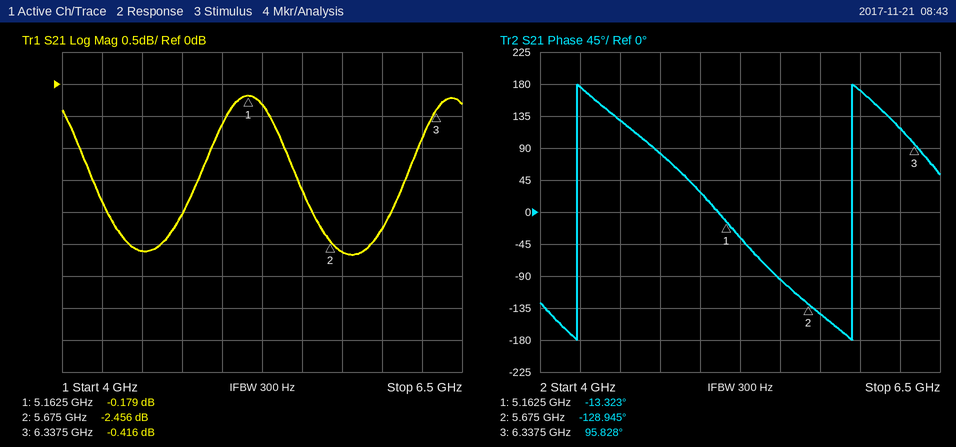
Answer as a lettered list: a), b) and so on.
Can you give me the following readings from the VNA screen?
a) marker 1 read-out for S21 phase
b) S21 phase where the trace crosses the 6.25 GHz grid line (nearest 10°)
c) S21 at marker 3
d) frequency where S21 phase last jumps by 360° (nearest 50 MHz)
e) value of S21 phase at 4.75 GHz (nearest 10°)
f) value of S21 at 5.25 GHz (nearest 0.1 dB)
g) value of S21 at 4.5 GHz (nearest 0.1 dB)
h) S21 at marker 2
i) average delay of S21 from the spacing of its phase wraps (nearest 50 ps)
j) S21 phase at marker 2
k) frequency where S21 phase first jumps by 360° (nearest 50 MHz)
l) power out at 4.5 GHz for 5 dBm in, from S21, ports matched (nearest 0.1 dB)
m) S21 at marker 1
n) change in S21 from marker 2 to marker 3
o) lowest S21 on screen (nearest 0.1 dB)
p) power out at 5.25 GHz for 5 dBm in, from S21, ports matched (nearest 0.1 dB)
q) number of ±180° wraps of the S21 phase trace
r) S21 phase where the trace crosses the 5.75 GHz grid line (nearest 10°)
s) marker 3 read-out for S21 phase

a) -13.323°
b) 120°
c) -0.416 dB
d) 5.95 GHz
e) 80°
f) -0.3 dB
g) -2.6 dB
h) -2.456 dB
i) 600 ps
j) -128.945°
k) 4.25 GHz
l) 2.4 dBm
m) -0.179 dB
n) 2.040 dB
o) -2.7 dB
p) 4.7 dBm
q) 2
r) -140°
s) 95.828°
